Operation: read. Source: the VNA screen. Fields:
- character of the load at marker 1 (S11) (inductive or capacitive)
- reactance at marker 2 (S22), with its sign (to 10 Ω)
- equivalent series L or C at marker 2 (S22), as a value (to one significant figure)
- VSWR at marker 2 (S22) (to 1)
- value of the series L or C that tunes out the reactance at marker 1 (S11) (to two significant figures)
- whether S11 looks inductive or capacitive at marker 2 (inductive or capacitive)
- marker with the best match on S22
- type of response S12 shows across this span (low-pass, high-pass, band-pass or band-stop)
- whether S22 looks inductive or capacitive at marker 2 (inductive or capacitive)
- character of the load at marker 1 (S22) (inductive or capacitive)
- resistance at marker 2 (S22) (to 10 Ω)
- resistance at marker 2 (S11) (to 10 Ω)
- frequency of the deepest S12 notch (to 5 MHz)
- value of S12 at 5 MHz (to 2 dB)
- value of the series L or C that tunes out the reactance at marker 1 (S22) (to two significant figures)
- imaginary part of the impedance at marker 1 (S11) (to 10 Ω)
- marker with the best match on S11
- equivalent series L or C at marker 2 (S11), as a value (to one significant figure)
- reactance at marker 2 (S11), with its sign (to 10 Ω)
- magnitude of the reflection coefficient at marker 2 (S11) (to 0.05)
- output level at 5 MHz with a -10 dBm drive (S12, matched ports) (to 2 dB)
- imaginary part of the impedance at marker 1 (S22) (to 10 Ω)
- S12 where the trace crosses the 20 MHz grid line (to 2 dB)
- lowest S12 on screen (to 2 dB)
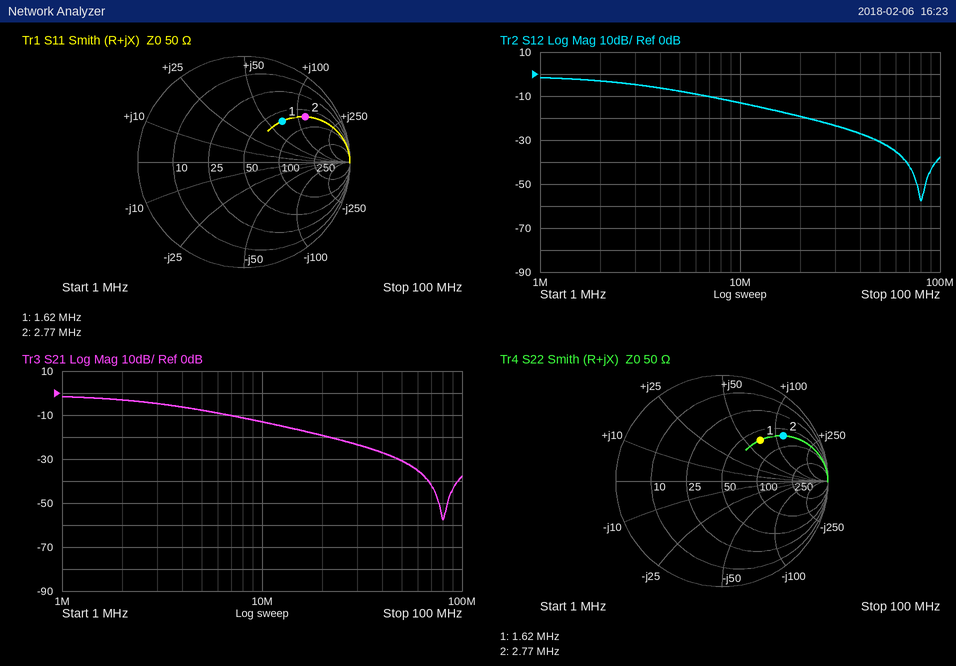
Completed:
inductive
+120 Ω
7 µH
6
1.4 nF
inductive
marker 1
low-pass
inductive
inductive
70 Ω
70 Ω
80 MHz
-8 dB
1.4 nF
+70 Ω
marker 1
7 µH
+120 Ω
0.70
-18 dBm
+70 Ω
-20 dB
-58 dB
